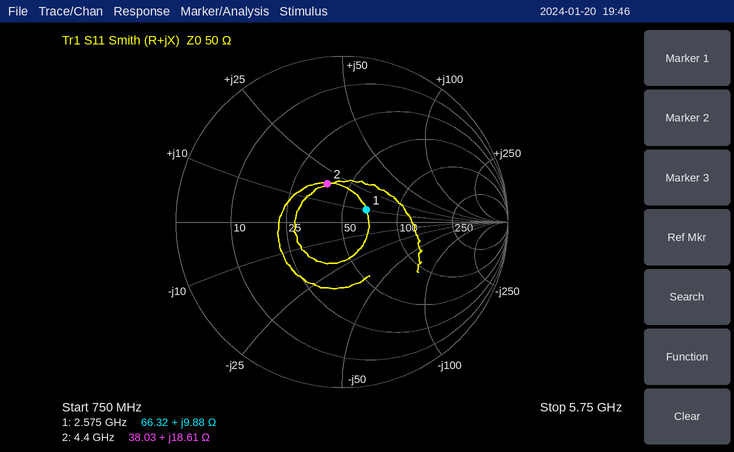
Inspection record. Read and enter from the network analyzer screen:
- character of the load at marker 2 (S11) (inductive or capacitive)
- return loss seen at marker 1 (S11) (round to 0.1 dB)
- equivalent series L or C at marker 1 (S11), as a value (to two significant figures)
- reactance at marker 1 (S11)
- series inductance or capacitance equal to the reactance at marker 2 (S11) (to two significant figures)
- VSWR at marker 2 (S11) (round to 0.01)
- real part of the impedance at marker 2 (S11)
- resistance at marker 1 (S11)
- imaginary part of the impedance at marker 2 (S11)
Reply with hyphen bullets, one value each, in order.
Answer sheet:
- inductive
- 15.7 dB
- 610 pH
- +9.88 Ω
- 670 pH
- 1.65
- 38.03 Ω
- 66.32 Ω
- +18.61 Ω
